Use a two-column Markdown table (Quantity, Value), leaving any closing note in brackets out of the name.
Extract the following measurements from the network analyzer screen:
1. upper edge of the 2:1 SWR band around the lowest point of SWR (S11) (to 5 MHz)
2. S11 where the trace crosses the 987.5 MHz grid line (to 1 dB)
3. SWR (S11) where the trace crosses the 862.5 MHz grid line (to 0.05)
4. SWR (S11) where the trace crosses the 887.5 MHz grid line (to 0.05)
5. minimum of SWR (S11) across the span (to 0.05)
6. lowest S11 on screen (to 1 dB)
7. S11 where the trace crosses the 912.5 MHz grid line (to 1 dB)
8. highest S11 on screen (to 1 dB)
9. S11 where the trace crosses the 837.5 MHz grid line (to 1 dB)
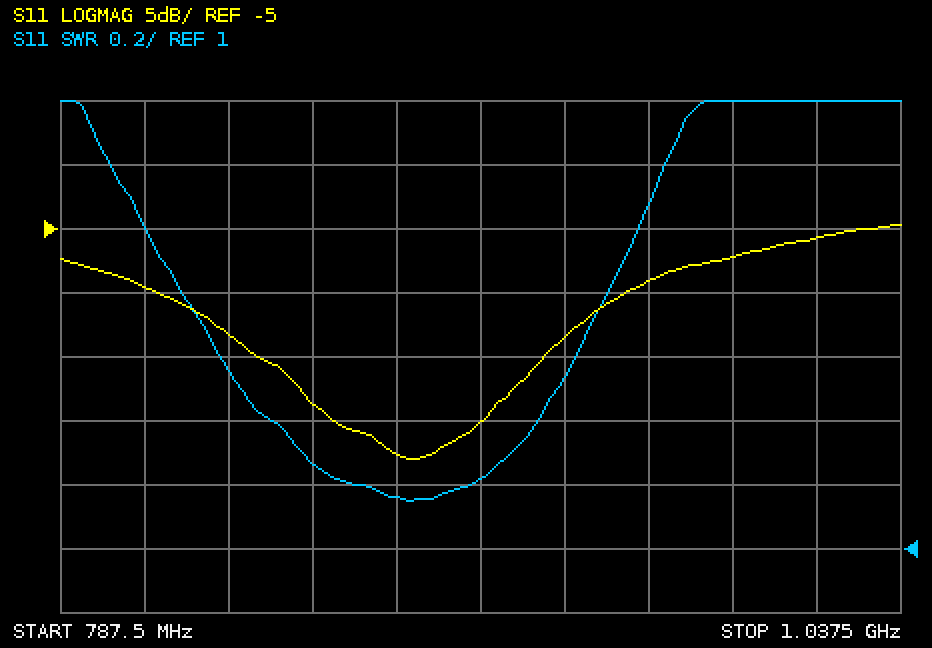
| Quantity | Value |
|---|---|
| upper edge of the 2:1 SWR band around the lowest point of SWR (S11) | 960 MHz |
| S11 where the trace crosses the 987.5 MHz grid line | -7 dB |
| SWR (S11) where the trace crosses the 862.5 MHz grid line | 1.25 |
| SWR (S11) where the trace crosses the 887.5 MHz grid line | 1.15 |
| minimum of SWR (S11) across the span | 1.15 |
| lowest S11 on screen | -23 dB |
| S11 where the trace crosses the 912.5 MHz grid line | -20 dB |
| highest S11 on screen | -5 dB |
| S11 where the trace crosses the 837.5 MHz grid line | -13 dB |
